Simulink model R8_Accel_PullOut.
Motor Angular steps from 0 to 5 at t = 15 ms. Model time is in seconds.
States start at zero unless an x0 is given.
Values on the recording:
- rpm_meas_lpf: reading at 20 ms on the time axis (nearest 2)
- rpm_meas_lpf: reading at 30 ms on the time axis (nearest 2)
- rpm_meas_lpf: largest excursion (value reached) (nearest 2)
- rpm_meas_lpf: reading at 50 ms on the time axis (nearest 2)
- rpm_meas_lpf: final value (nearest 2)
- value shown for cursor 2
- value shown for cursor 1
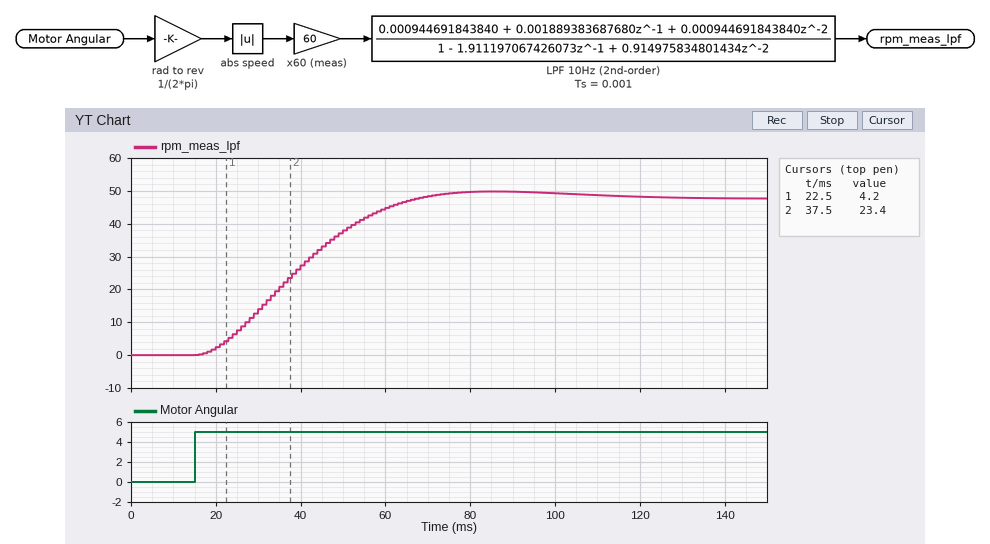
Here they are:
2
14
50
38
48
23.4
4.2
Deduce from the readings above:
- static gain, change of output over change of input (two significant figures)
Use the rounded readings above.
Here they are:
9.6
